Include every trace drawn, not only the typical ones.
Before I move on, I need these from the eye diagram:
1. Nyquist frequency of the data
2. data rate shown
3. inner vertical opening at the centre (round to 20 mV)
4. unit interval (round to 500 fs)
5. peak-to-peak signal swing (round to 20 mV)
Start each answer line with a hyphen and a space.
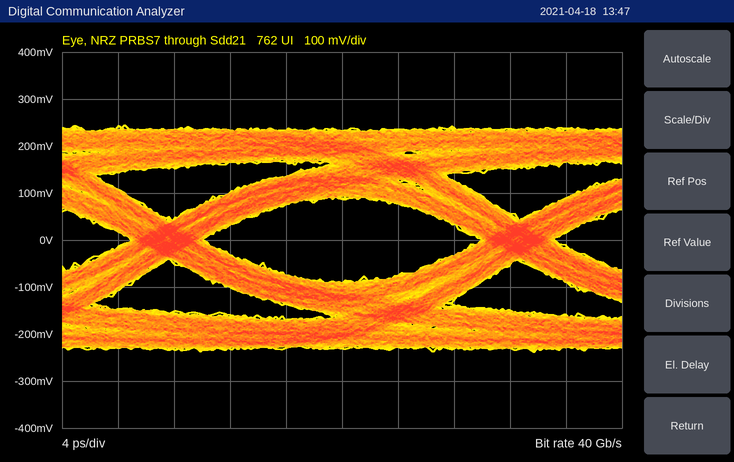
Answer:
- 20 GHz
- 40 Gb/s
- 180 mV
- 25.0 ps
- 480 mV
